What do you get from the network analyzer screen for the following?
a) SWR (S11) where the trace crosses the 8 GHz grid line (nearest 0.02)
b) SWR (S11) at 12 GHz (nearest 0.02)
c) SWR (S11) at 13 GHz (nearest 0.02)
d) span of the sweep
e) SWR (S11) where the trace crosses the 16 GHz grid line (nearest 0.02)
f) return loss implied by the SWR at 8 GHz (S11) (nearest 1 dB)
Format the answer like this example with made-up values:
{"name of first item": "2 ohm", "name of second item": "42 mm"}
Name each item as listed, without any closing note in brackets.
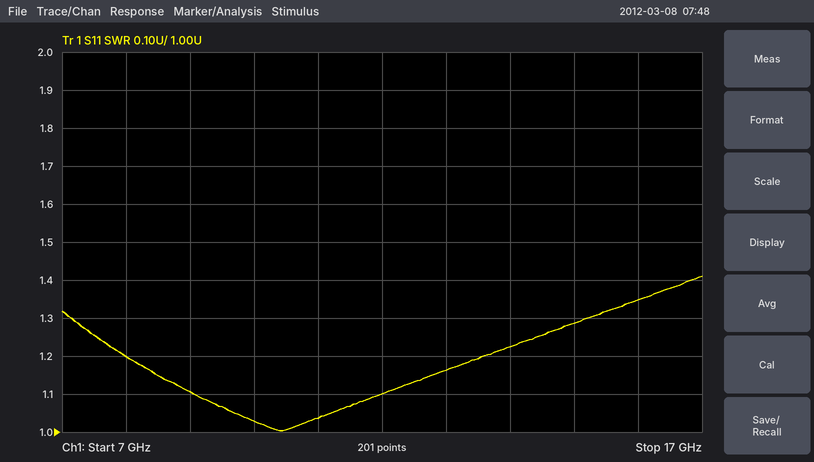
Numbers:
{"SWR (S11) where the trace crosses the 8 GHz grid line": "1.20", "SWR (S11) at 12 GHz": "1.10", "SWR (S11) at 13 GHz": "1.16", "span of the sweep": "10 GHz", "SWR (S11) where the trace crosses the 16 GHz grid line": "1.34", "return loss implied by the SWR at 8 GHz (S11)": "21 dB"}
